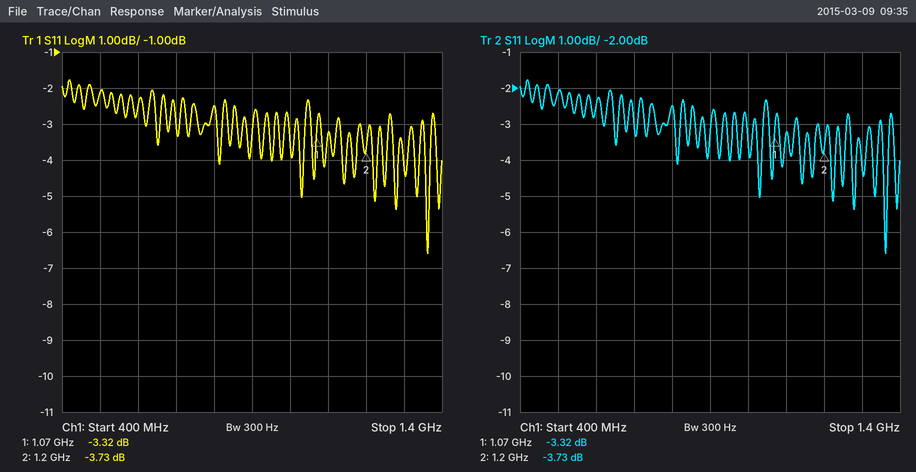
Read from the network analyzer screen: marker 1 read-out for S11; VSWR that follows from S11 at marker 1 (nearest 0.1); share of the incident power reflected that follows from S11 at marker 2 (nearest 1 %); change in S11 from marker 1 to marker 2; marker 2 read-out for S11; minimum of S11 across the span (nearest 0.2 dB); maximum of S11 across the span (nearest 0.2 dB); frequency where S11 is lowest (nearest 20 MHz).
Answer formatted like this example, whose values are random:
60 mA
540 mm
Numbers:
-3.32 dB
5.3
42 %
-0.41 dB
-3.73 dB
-6.6 dB
-1.8 dB
1.36 GHz
